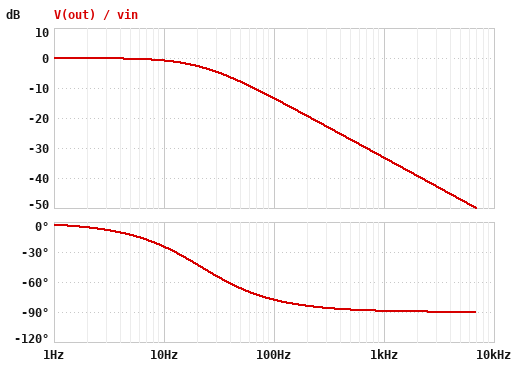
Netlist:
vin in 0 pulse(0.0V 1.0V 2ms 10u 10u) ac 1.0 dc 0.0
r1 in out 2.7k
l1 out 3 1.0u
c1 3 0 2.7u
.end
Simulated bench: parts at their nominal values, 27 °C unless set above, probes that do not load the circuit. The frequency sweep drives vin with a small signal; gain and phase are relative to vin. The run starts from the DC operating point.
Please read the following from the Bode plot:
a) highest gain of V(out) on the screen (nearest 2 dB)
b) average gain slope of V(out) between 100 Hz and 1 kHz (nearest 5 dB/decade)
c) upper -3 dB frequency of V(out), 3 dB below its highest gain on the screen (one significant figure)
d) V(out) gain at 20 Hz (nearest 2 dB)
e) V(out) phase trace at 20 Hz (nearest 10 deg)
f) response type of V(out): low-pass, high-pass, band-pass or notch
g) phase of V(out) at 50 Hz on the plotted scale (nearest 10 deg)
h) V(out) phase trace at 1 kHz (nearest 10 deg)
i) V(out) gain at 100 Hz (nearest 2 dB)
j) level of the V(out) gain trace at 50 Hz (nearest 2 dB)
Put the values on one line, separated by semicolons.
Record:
0 dB; -20 dB/decade; 20 Hz; -2 dB; -40 deg; low-pass; -70 deg; -90 deg; -14 dB; -8 dB
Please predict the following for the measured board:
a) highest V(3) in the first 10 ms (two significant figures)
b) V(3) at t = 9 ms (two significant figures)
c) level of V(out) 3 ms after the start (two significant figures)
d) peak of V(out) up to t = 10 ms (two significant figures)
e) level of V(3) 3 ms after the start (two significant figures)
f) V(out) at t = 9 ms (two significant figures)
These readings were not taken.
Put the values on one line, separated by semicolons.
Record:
670 mV; 620 mV; 130 mV; 670 mV; 130 mV; 620 mV
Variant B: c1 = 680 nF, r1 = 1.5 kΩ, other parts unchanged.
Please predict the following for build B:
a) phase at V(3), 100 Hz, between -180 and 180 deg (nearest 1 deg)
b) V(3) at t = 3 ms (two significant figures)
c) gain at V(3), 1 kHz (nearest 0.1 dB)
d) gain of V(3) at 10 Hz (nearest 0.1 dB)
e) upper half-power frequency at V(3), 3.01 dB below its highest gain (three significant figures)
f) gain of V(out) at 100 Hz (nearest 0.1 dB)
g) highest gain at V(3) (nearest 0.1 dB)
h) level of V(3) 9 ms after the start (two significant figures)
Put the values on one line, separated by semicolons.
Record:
-33 deg; 620 mV; -16.2 dB; 0 dB; 156 Hz; -1.5 dB; 0 dB; 1.0 V
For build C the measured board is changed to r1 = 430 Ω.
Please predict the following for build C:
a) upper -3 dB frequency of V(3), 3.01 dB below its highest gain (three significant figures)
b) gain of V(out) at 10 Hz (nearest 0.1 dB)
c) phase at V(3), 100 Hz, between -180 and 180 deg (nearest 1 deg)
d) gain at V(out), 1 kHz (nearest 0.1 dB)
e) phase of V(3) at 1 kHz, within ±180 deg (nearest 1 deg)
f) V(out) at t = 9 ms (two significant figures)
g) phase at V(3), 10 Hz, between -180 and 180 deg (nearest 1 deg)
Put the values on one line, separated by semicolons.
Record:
137 Hz; 0 dB; -36 deg; -17.3 dB; -82 deg; 1.0 V; -4 deg
